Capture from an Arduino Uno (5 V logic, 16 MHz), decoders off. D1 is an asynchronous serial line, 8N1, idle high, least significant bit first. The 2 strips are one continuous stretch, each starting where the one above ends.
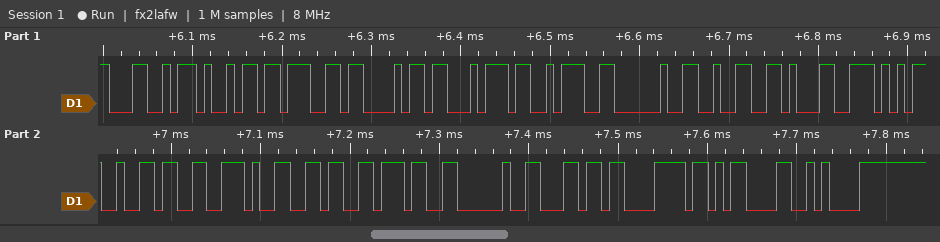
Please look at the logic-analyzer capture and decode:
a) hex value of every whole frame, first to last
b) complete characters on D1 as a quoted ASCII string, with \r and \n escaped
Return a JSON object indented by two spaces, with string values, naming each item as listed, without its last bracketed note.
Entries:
{
  "hex value of every whole frame, first to last": "4C 69 67 68 74 3A 20 32 31 35 36 2E 36 37 20 6C 78 0D 0A",
  "complete characters on D1 as a quoted ASCII string, with \\r and \\n escaped": "\"Light: 2156.67 lx\\r\\n\""
}
